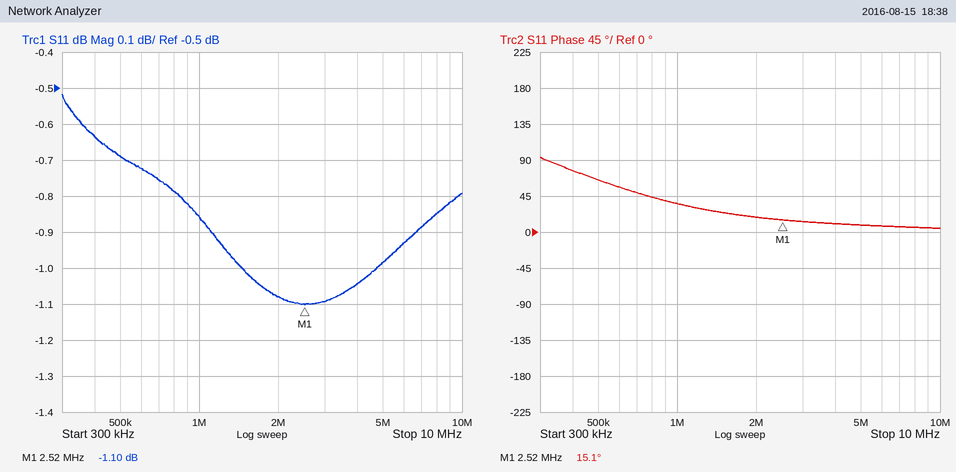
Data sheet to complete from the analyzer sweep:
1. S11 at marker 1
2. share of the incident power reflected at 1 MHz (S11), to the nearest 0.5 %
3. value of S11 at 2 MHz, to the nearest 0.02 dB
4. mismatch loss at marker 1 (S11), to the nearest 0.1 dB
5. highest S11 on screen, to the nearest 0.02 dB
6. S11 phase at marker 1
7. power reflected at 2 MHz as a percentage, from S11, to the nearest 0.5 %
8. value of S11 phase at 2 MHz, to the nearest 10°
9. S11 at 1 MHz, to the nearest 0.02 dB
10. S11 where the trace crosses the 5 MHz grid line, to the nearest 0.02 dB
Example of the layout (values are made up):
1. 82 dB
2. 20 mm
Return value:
1. -1.10 dB
2. 82.0 %
3. -1.08 dB
4. 6.5 dB
5. -0.52 dB
6. 15.1°
7. 78.0 %
8. 20°
9. -0.86 dB
10. -0.98 dB
